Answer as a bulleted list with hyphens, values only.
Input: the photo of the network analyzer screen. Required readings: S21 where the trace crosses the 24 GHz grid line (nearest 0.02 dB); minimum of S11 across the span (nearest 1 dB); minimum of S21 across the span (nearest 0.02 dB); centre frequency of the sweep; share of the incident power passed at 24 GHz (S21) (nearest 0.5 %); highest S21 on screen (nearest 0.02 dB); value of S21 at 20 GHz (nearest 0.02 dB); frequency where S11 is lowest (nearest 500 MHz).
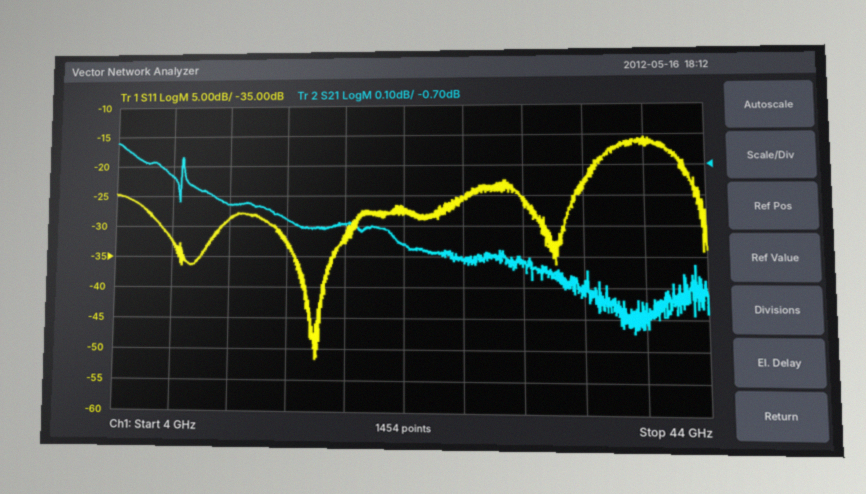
- -0.96 dB
- -52 dB
- -1.24 dB
- 24 GHz
- 80.0 %
- -0.62 dB
- -0.90 dB
- 18.0 GHz
